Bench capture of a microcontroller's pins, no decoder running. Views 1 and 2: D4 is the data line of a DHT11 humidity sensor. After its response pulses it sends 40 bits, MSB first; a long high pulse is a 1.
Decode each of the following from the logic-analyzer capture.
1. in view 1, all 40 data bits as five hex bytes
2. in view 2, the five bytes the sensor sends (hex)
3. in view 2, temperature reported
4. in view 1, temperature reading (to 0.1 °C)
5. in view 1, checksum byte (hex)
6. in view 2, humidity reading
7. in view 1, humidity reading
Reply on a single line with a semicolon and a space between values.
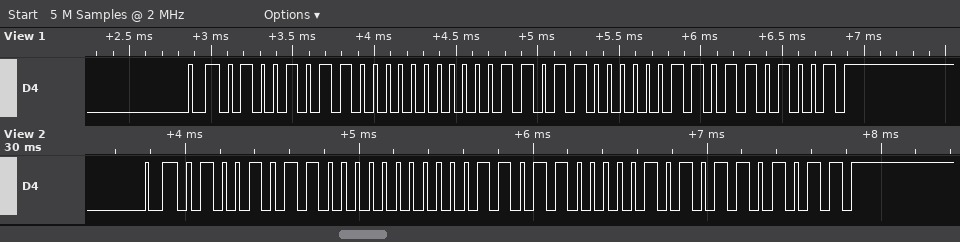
4B 00 1B 03 69; 4B 00 1B 05 6B; 27.5 °C; 27.3 °C; 0x69; 75 %; 75 %
